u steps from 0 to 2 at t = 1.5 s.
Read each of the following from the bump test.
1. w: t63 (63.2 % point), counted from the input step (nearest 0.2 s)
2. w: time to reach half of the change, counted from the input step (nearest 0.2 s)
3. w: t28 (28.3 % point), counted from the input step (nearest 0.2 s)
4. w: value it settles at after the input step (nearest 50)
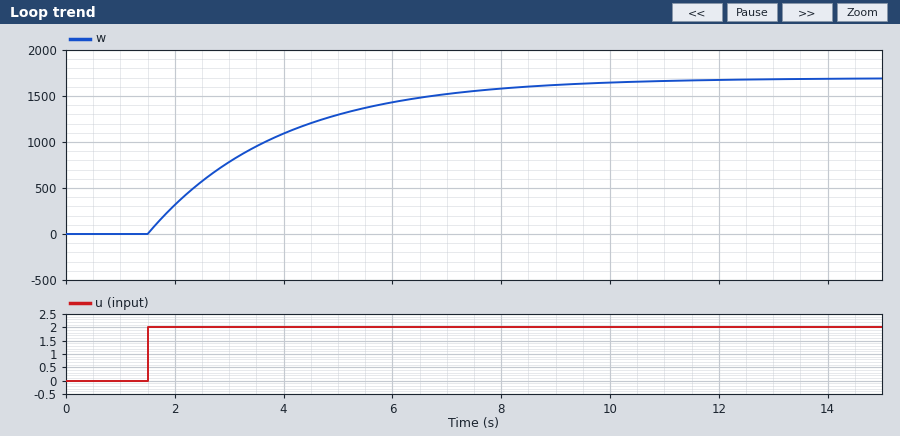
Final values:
2.4 s
1.6 s
0.8 s
1700
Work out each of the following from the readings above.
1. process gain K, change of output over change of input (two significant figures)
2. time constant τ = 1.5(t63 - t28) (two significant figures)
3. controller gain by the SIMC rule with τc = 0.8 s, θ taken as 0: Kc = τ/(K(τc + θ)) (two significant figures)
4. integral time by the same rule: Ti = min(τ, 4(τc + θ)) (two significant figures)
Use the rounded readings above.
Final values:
850
2.4 s
0.0035
2.4 s
